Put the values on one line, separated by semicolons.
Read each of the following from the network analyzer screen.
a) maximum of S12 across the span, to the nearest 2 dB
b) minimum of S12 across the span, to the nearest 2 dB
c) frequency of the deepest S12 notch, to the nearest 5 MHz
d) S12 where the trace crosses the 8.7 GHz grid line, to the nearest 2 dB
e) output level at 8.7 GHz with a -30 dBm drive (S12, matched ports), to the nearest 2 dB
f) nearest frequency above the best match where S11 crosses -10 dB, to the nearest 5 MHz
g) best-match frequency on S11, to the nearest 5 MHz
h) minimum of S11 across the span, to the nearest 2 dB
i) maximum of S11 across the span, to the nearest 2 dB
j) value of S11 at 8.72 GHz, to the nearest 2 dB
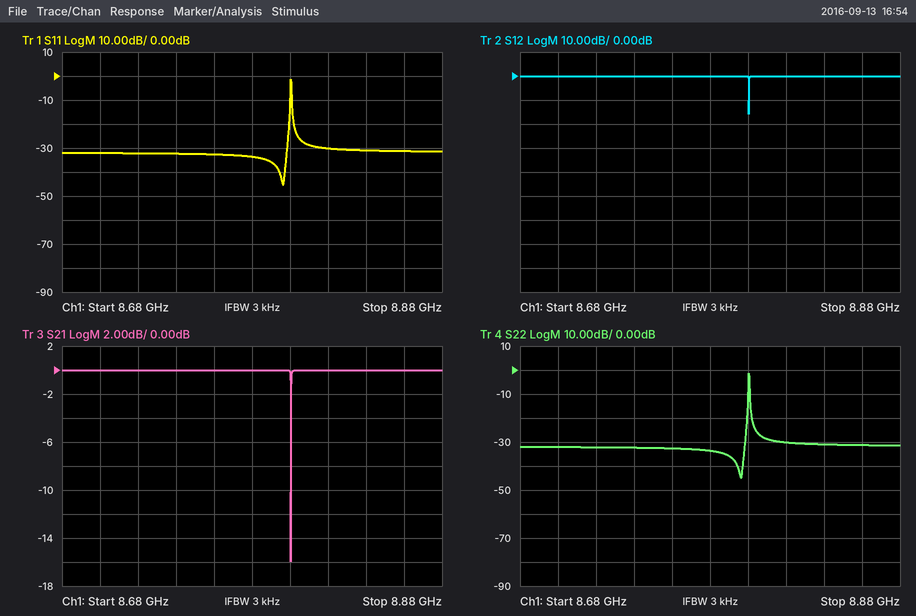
0 dB; -16 dB; 8.800 GHz; 0 dB; -30 dBm; 8.800 GHz; 8.795 GHz; -46 dB; -2 dB; -32 dB
